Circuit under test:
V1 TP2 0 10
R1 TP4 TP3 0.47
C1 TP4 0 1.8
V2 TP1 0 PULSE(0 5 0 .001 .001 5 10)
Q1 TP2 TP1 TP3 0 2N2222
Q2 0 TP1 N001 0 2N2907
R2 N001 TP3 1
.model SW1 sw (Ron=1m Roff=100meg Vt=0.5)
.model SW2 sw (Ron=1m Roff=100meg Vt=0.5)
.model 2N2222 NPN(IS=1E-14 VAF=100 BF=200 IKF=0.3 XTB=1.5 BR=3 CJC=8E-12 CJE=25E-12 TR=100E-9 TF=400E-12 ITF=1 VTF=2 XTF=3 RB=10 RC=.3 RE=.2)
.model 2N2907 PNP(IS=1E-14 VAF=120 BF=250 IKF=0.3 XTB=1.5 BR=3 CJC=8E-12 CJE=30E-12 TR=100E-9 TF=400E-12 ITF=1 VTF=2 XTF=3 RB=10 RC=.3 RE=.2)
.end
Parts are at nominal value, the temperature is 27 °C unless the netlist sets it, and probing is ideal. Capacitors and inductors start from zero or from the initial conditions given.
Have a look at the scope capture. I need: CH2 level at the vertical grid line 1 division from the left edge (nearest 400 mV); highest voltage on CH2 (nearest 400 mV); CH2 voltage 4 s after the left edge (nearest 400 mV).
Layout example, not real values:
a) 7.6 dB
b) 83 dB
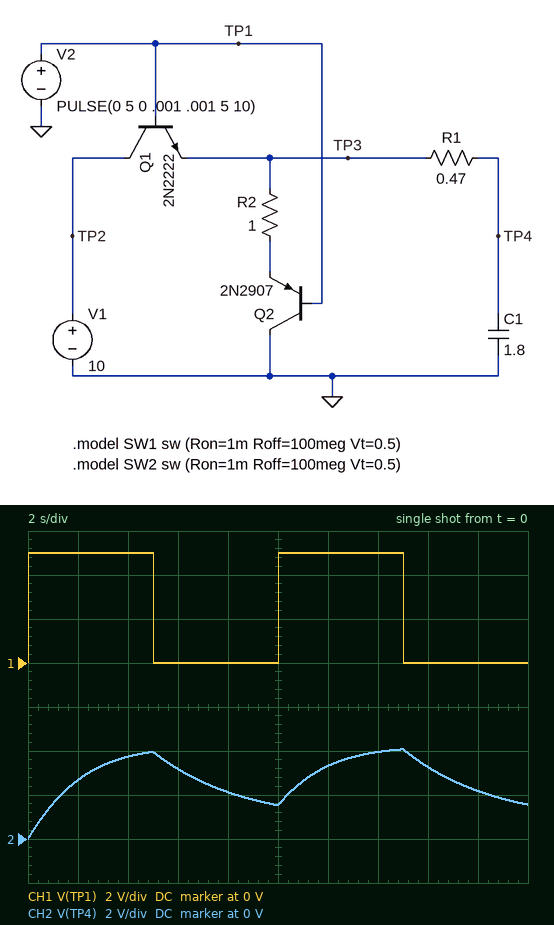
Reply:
a) 2.8 V
b) 4.0 V
c) 3.6 V
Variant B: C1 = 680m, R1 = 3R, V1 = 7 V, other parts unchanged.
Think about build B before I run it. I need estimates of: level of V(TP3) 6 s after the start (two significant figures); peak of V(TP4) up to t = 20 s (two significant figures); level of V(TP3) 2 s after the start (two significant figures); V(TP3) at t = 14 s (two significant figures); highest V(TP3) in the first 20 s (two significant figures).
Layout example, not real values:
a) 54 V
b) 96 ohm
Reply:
a) 1.5 V
b) 3.9 V
c) 4.0 V
d) 4.2 V
e) 4.2 V
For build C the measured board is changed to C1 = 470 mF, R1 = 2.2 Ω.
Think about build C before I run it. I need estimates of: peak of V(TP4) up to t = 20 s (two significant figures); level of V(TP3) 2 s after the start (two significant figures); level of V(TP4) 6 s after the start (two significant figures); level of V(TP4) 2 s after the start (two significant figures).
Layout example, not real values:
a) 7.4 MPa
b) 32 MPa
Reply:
a) 4.2 V
b) 4.1 V
c) 2.7 V
d) 3.4 V
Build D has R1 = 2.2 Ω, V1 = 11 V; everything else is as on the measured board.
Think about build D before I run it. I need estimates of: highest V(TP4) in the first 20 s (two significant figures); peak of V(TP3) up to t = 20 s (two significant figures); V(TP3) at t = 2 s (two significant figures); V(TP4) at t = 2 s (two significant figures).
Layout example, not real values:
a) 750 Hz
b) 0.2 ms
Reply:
a) 3.3 V
b) 4.1 V
c) 3.7 V
d) 1.4 V
